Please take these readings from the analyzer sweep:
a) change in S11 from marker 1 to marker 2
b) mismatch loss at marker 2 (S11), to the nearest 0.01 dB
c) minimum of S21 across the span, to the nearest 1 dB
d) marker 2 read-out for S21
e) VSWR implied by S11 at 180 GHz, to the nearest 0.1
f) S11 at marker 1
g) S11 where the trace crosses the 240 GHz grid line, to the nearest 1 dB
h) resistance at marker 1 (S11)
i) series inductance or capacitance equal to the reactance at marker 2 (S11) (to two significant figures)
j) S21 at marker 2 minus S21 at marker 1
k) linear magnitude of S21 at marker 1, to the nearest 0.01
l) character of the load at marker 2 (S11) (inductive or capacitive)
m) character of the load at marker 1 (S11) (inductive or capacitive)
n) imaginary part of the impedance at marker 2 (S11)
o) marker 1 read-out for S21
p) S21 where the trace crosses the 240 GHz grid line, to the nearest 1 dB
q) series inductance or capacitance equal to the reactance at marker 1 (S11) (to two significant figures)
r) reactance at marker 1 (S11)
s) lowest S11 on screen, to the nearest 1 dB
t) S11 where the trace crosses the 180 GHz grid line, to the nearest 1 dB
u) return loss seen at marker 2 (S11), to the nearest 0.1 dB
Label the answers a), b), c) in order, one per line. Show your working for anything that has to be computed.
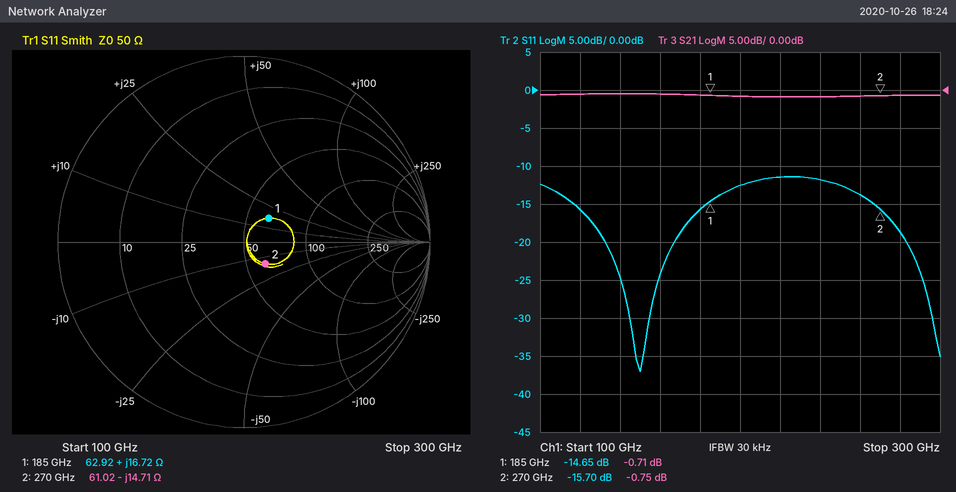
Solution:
a) -15.7 − (-14.65) = -1.05 dB
b) −10 log10(1 − 10^(-15.7/10)) ≈ 0.12 dB
c) -1 dB
d) -0.75 dB
e) |Γ| = 10^(-16/20) = 0.1585; VSWR = (1 + 0.1585)/(1 − 0.1585) ≈ 1.4
f) -14.65 dB
g) -12 dB
h) 62.92 Ω
i) C = 1/(2π × 270 GHz × 14.71 Ω) ≈ 40 fF
j) -0.75 − (-0.71) = -0.04 dB
k) 10^(-0.71/20) ≈ 0.92
l) capacitive
m) inductive
n) -14.71 Ω
o) -0.71 dB
p) -1 dB
q) L = 16.72 Ω/(2π × 185 GHz) ≈ 14 pH
r) +16.72 Ω
s) -37 dB
t) -16 dB
u) 15.7 dB
